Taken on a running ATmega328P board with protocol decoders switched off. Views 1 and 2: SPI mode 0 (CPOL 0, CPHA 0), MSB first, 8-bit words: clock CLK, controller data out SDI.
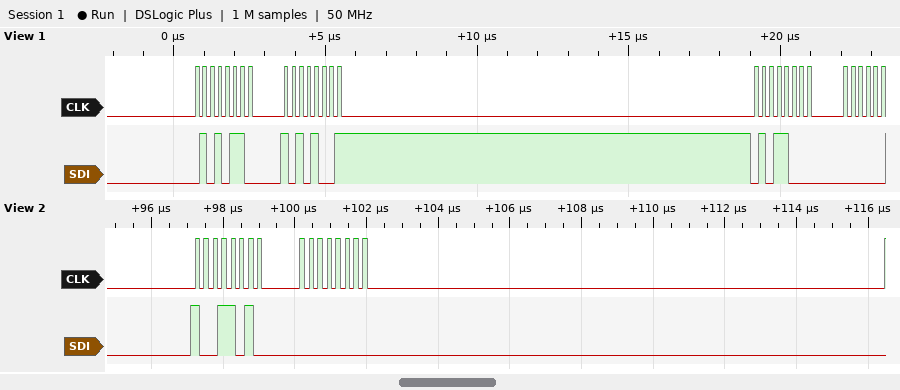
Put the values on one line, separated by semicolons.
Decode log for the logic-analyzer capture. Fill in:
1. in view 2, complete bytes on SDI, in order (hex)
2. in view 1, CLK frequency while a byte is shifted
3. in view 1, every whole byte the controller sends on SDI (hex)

9A 00; 4 MHz; 56 A9 58
